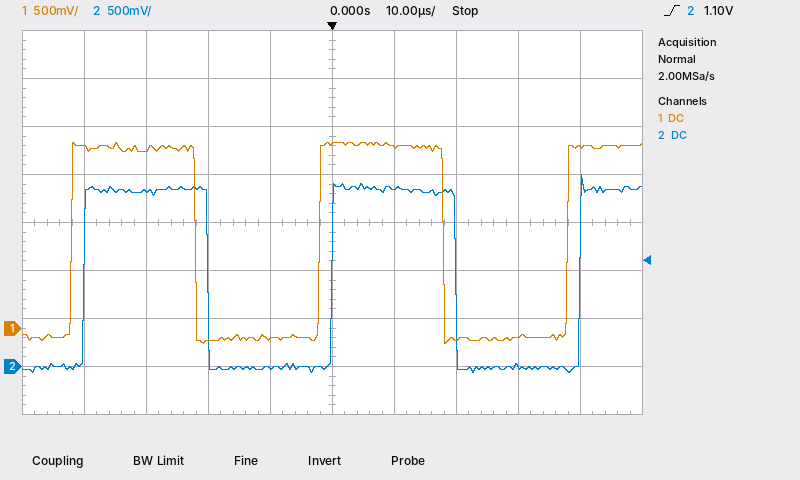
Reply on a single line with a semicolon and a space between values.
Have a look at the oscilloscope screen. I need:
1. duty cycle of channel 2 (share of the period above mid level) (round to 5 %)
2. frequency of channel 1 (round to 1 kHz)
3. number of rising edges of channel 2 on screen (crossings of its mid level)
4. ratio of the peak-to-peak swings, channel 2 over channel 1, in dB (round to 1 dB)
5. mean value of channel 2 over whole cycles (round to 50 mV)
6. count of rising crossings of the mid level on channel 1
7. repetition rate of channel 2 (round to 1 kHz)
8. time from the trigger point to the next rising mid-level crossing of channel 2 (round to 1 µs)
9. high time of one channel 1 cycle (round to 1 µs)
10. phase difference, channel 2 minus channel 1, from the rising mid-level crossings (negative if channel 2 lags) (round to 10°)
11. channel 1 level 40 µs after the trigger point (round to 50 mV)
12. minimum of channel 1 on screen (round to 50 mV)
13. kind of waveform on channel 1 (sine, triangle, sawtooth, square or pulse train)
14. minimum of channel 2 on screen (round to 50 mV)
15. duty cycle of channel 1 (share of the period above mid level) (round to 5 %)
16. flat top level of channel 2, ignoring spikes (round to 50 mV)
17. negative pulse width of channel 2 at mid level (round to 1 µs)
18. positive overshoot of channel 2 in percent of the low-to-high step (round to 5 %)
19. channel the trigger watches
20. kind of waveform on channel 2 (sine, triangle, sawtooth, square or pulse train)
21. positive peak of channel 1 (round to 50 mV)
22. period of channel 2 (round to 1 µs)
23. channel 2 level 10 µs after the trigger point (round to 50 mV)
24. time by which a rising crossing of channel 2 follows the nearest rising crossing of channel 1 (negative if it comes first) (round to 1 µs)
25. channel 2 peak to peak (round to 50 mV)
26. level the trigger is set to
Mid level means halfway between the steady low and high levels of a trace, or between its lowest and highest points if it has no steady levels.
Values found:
50 %; 25 kHz; 3; 0 dB; 900 mV; 3; 25 kHz; 40 µs; 20 µs; -20°; 1.90 V; -150 mV; square; -50 mV; 50 %; 1.85 V; 20 µs; 10 %; channel 2; square; 1.95 V; 40 µs; 1.85 V; +2 µs; 2.05 V; 1.10 V
